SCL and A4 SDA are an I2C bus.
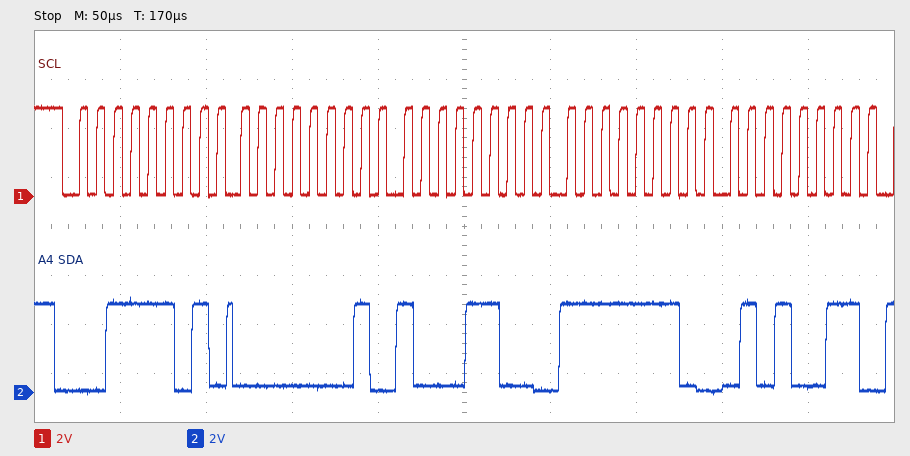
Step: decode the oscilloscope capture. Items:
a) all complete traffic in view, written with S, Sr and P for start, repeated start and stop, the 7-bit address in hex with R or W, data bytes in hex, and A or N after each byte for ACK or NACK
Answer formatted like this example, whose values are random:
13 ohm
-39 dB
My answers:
S 1ER A 01 A 8C A FE A 53 A
